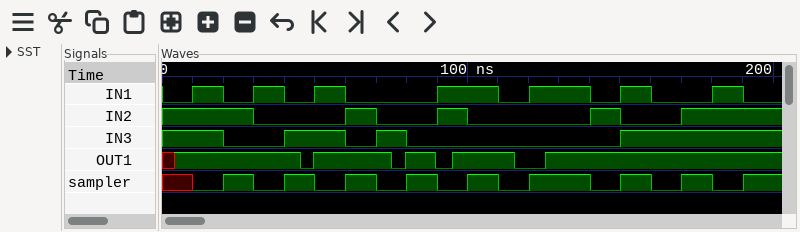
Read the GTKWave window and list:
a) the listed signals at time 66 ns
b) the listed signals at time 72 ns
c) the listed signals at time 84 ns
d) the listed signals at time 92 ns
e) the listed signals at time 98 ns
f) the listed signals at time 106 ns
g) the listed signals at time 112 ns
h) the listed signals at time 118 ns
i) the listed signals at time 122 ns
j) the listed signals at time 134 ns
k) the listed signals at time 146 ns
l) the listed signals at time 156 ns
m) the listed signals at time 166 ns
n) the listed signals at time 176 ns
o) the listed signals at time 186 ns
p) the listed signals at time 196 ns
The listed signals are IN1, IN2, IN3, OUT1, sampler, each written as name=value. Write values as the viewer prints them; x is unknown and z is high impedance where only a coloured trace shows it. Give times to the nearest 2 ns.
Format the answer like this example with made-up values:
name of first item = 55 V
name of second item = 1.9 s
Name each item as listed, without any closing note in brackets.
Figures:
the listed signals at time 66 ns = IN1=0, IN2=1, IN3=0, OUT1=1, sampler=1
the listed signals at time 72 ns = IN1=0, IN2=0, IN3=1, OUT1=1, sampler=0
the listed signals at time 84 ns = IN1=0, IN2=0, IN3=0, OUT1=1, sampler=1
the listed signals at time 92 ns = IN1=1, IN2=1, IN3=0, OUT1=0, sampler=0
the listed signals at time 98 ns = IN1=1, IN2=1, IN3=0, OUT1=1, sampler=0
the listed signals at time 106 ns = IN1=1, IN2=0, IN3=0, OUT1=1, sampler=1
the listed signals at time 112 ns = IN1=0, IN2=0, IN3=0, OUT1=1, sampler=0
the listed signals at time 118 ns = IN1=0, IN2=0, IN3=0, OUT1=0, sampler=0
the listed signals at time 122 ns = IN1=1, IN2=0, IN3=0, OUT1=0, sampler=1
the listed signals at time 134 ns = IN1=1, IN2=0, IN3=0, OUT1=1, sampler=1
the listed signals at time 146 ns = IN1=0, IN2=1, IN3=0, OUT1=1, sampler=0
the listed signals at time 156 ns = IN1=1, IN2=0, IN3=1, OUT1=1, sampler=1
the listed signals at time 166 ns = IN1=0, IN2=0, IN3=1, OUT1=1, sampler=0
the listed signals at time 176 ns = IN1=0, IN2=1, IN3=1, OUT1=1, sampler=1
the listed signals at time 186 ns = IN1=1, IN2=1, IN3=1, OUT1=1, sampler=0
the listed signals at time 196 ns = IN1=0, IN2=1, IN3=1, OUT1=1, sampler=1
